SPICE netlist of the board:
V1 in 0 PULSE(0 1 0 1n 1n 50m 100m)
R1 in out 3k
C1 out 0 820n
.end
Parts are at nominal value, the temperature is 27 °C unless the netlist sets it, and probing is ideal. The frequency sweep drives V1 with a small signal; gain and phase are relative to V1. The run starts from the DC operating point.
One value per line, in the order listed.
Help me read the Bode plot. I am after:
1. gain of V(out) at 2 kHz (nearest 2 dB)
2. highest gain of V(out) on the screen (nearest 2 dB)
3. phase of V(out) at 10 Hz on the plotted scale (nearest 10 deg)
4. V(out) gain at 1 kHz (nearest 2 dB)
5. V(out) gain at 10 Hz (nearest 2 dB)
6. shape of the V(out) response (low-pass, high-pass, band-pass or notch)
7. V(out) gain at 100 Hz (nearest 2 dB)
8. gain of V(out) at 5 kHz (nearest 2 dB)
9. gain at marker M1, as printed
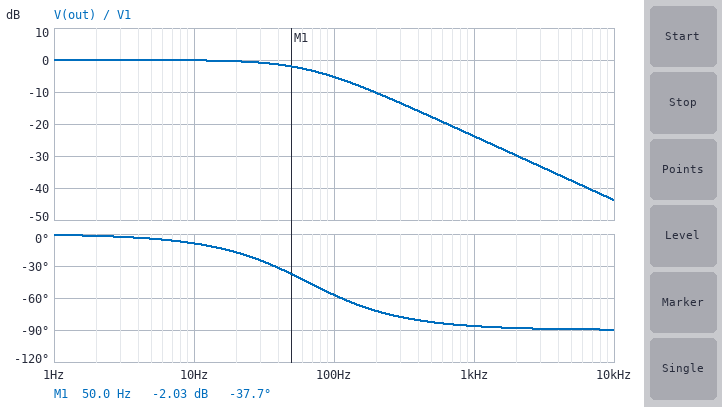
-30 dB
0 dB
-10 deg
-24 dB
0 dB
low-pass
-6 dB
-38 dB
-2.03 dB
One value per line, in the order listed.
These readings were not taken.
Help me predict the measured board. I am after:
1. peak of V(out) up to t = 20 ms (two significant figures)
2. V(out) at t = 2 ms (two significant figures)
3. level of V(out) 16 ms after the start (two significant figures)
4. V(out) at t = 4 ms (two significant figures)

1.0 V
560 mV
1.0 V
800 mV
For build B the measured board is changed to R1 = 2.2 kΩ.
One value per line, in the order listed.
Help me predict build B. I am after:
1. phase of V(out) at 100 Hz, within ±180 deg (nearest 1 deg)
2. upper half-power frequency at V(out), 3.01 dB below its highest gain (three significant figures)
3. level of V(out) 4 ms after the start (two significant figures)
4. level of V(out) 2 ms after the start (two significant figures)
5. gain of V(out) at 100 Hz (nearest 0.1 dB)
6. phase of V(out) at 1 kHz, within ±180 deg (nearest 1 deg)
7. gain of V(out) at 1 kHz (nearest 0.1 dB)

-49 deg
88.2 Hz
890 mV
670 mV
-3.6 dB
-85 deg
-21.1 dB
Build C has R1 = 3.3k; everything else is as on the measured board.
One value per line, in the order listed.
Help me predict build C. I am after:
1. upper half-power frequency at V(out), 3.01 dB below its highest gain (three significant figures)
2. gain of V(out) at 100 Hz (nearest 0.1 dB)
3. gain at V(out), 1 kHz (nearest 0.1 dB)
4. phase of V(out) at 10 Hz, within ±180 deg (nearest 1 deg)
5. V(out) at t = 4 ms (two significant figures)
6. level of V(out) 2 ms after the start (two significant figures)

58.8 Hz
-5.9 dB
-24.6 dB
-10 deg
770 mV
520 mV
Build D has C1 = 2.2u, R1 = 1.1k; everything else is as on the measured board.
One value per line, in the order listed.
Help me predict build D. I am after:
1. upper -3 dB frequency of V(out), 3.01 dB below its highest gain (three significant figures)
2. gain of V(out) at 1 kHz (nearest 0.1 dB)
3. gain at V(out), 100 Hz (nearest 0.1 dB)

65.8 Hz
-23.7 dB
-5.2 dB
